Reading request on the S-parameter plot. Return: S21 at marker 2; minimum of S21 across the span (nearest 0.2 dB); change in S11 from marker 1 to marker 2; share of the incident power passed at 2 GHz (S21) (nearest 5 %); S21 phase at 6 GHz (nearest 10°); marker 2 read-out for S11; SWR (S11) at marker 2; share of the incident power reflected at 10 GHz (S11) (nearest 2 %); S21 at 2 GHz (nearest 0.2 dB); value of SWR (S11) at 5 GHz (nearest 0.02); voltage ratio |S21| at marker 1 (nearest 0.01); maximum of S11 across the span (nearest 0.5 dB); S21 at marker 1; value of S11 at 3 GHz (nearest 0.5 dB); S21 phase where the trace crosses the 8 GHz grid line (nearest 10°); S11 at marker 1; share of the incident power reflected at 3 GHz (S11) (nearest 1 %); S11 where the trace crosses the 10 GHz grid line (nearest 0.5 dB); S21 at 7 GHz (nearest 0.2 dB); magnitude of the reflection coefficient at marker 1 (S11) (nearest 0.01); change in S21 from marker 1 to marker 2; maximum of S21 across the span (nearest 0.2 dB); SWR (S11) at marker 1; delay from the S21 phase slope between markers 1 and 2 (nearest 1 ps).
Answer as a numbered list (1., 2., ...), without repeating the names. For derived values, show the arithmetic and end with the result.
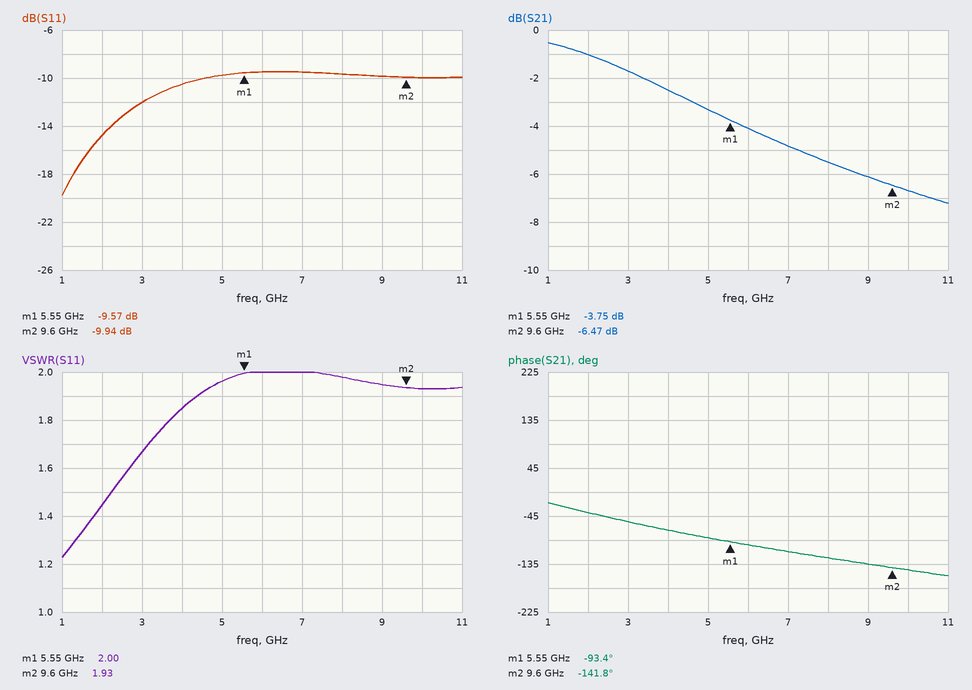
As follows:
1. -6.47 dB
2. -7.2 dB
3. -9.94 − (-9.57) = -0.37 dB
4. 10^(-1/10) ≈ 79.4 %, so 80 % to the nearest 5 %
5. -100°
6. -9.94 dB
7. 1.93
8. 10^(-10/10) ≈ 10 %
9. -1.0 dB
10. 1.96
11. 10^(-3.75/20) ≈ 0.65
12. -9.5 dB
13. -3.75 dB
14. -12.0 dB
15. -120°
16. -9.57 dB
17. 10^(-12/10) ≈ 6 %
18. -10.0 dB
19. -4.8 dB
20. 10^(-9.57/20) ≈ 0.33
21. -6.47 − (-3.75) = -2.72 dB
22. -0.6 dB
23. 2.00
24. −(-141.8° − (-93.4°))/(360° × 4.05 GHz) ≈ 33 ps
